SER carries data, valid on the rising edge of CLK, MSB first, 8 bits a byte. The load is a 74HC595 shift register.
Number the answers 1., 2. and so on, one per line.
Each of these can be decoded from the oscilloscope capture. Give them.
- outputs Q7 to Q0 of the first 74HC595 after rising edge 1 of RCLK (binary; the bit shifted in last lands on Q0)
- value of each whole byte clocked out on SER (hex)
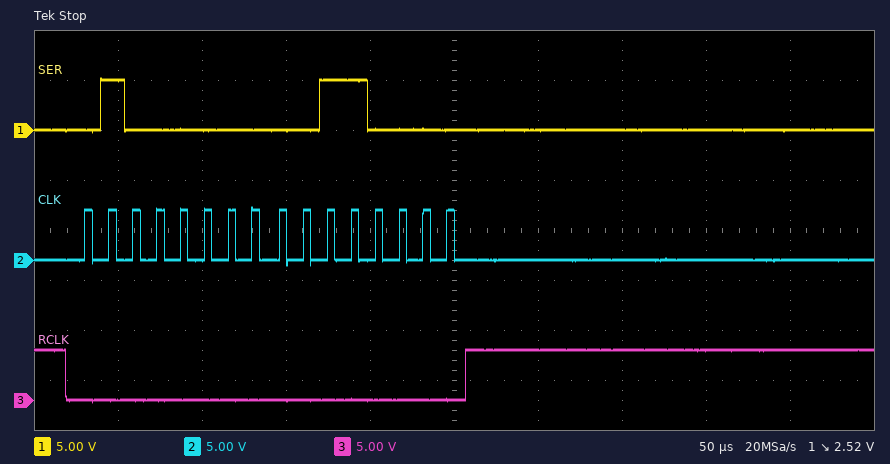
1. 00110000
2. 40 30
